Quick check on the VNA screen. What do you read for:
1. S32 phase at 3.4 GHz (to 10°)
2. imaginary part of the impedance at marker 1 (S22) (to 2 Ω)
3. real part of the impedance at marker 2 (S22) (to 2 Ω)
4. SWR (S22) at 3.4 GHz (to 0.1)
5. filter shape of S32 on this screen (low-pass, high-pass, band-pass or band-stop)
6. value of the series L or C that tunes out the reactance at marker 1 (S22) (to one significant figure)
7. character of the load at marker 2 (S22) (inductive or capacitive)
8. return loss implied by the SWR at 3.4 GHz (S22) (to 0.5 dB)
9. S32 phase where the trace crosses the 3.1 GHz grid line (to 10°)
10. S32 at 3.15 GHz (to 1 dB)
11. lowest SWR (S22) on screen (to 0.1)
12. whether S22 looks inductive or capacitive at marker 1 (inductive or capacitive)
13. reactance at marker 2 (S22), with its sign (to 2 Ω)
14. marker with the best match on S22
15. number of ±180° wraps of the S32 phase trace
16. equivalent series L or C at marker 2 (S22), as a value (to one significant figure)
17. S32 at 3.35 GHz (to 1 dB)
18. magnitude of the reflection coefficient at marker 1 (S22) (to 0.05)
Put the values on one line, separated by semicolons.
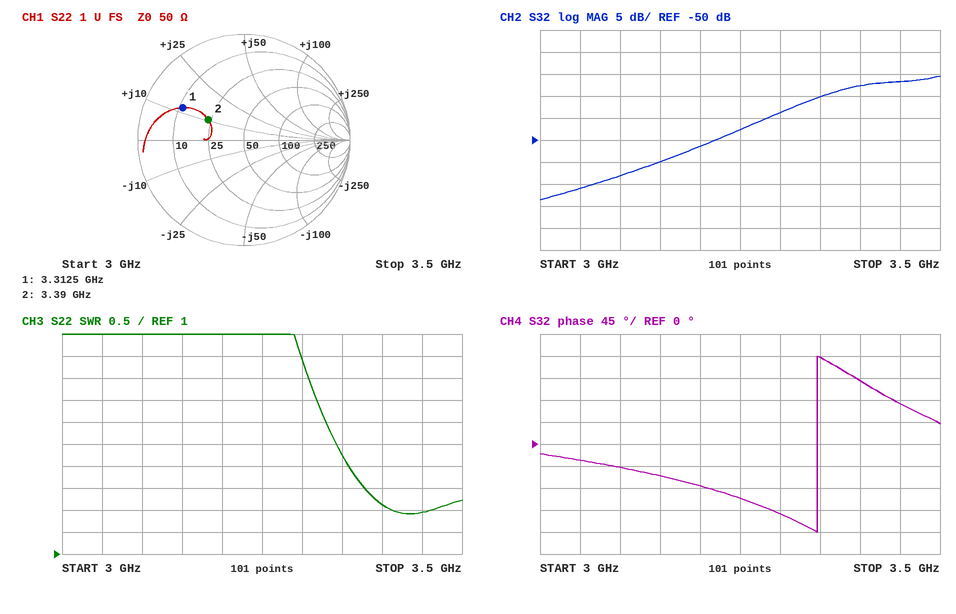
130°; +12 Ω; 24 Ω; 2.1; high-pass; 4 pF; inductive; 9.0 dB; -50°; -55 dB; 1.9; inductive; +10 Ω; marker 2; 1; 500 pH; -40 dB; 0.65
